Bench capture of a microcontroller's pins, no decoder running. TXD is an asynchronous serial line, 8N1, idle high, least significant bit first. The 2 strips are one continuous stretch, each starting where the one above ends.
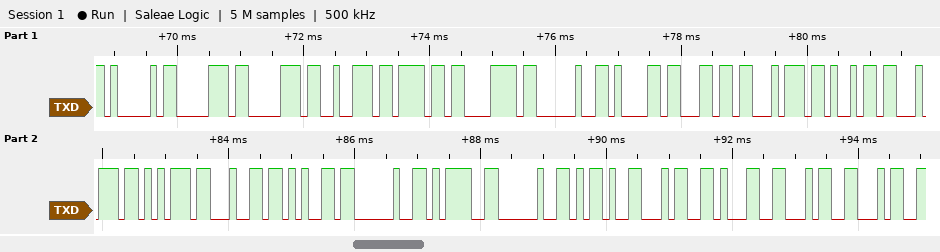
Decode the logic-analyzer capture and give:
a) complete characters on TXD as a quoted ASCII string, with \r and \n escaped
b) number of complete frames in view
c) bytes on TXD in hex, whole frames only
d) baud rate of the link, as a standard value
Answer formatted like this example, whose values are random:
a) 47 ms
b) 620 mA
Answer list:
a) "Approx altitude = -4144"
b) 23
c) 41 70 70 72 6F 78 20 61 6C 74 69 74 75 64 65 20 3D 20 2D 34 31 34 34
d) 9600 baud
